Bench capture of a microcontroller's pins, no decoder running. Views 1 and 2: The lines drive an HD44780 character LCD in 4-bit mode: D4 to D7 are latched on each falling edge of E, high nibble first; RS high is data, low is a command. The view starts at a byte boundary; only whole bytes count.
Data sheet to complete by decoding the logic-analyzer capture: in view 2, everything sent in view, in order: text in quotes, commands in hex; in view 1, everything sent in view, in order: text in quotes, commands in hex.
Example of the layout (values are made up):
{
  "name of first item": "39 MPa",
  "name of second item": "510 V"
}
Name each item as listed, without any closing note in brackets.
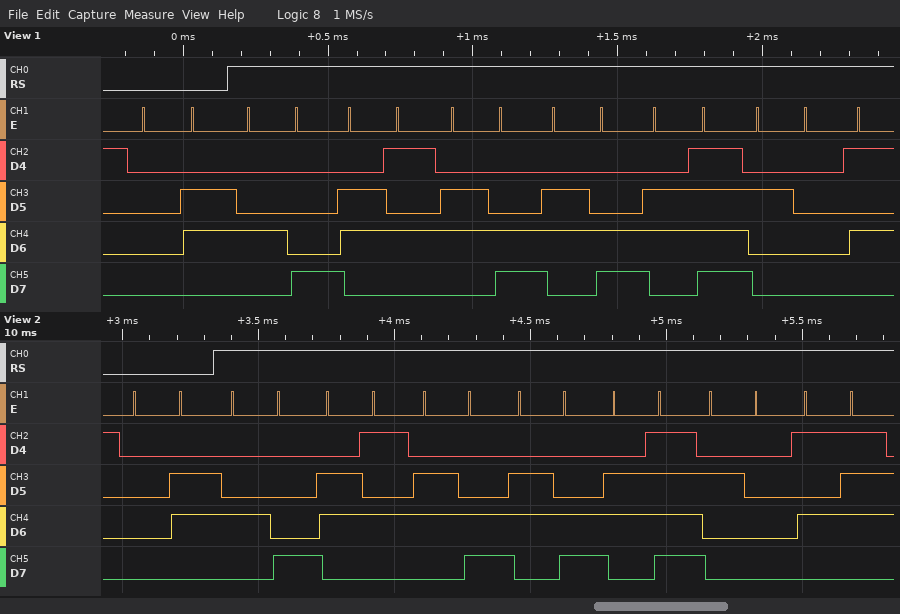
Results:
{
  "in view 2, everything sent in view, in order: text in quotes, commands in hex": "0x06 \"Hello W\"",
  "in view 1, everything sent in view, in order: text in quotes, commands in hex": "0x06 \"Hello \""
}
